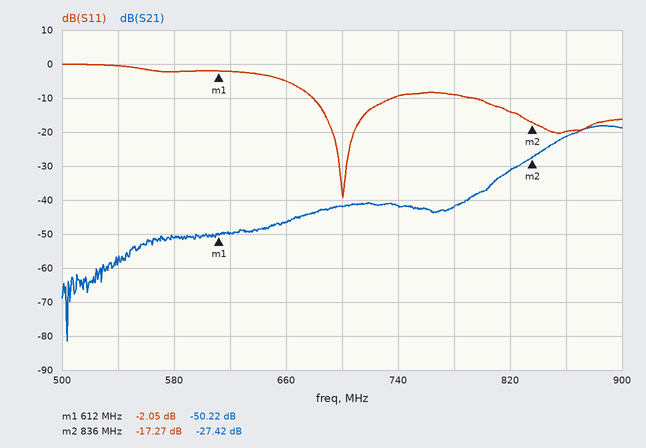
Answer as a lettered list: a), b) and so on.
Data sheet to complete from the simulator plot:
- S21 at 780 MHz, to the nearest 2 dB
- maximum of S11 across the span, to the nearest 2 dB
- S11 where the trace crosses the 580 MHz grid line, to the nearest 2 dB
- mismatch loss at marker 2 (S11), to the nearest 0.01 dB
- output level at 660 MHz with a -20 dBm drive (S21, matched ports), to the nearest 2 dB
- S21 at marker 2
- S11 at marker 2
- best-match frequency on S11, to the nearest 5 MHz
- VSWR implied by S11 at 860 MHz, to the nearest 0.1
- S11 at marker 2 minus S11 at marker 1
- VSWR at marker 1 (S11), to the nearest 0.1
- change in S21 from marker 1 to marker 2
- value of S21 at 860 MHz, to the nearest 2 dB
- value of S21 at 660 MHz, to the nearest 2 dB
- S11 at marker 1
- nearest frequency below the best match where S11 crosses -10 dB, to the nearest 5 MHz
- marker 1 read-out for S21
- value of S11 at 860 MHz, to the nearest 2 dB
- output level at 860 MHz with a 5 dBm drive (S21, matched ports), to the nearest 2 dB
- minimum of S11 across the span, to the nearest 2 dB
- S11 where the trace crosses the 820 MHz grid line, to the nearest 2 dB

a) -42 dB
b) 0 dB
c) -2 dB
d) 0.08 dB
e) -66 dBm
f) -27.42 dB
g) -17.27 dB
h) 700 MHz
i) 1.2
j) -15.22 dB
k) 8.5
l) 22.80 dB
m) -22 dB
n) -46 dB
o) -2.05 dB
p) 680 MHz
q) -50.22 dB
r) -20 dB
s) -16 dBm
t) -40 dB
u) -14 dB
